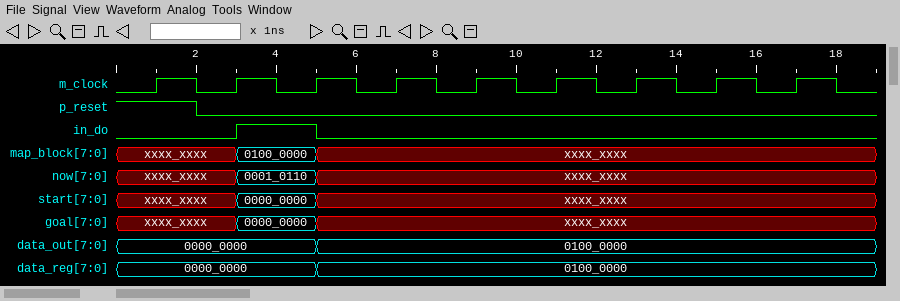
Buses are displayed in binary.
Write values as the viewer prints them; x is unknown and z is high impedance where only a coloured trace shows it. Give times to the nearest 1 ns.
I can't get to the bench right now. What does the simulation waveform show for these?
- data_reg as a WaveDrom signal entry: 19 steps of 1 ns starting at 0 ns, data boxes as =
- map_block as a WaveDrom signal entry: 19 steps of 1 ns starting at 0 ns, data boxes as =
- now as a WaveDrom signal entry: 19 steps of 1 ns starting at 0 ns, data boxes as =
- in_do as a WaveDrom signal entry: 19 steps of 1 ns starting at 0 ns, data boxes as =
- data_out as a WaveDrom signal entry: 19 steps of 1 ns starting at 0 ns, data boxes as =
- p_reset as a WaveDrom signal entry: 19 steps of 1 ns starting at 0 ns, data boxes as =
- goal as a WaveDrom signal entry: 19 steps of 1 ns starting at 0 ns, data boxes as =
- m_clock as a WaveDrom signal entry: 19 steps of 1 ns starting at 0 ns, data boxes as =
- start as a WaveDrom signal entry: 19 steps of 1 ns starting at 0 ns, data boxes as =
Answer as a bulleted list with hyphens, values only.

- {name: 'data_reg', wave: '=....=.............', data: '0000_0000 0100_0000'}
- {name: 'map_block', wave: 'x..=.x.............', data: '0100_0000'}
- {name: 'now', wave: 'x..=.x.............', data: '0001_0110'}
- {name: 'in_do', wave: '0..1.0.............'}
- {name: 'data_out', wave: '=....=.............', data: '0000_0000 0100_0000'}
- {name: 'p_reset', wave: '1.0................'}
- {name: 'goal', wave: 'x..=.x.............', data: '0000_0000'}
- {name: 'm_clock', wave: '0101010101010101010'}
- {name: 'start', wave: 'x..=.x.............', data: '0000_0000'}
